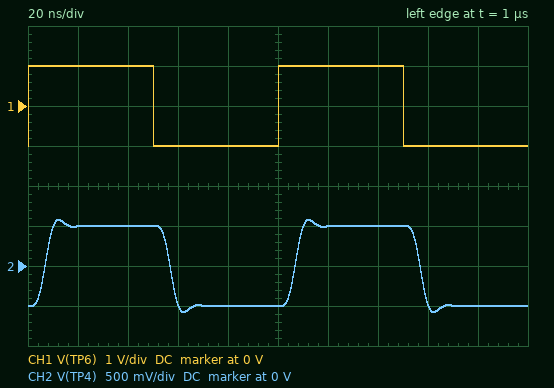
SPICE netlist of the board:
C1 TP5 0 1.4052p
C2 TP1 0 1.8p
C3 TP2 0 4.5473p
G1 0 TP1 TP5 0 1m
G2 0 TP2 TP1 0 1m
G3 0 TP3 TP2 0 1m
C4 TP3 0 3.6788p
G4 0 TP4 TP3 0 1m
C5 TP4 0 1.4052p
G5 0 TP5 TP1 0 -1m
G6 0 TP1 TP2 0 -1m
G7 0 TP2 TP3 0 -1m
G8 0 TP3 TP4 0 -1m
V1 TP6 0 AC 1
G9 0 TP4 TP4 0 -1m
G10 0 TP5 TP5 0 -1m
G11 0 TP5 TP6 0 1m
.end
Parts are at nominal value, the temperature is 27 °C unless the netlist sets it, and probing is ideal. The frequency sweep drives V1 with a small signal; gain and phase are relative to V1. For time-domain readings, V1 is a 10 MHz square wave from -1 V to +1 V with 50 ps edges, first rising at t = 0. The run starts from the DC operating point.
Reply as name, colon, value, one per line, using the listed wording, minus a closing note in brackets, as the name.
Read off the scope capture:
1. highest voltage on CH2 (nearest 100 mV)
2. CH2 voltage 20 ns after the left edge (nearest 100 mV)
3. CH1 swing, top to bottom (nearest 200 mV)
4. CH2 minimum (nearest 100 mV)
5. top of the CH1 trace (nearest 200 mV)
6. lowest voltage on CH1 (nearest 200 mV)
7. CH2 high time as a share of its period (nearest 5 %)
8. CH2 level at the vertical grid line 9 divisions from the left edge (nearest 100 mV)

highest voltage on CH2: 600 mV
CH2 voltage 20 ns after the left edge: 500 mV
CH1 swing, top to bottom: 2.0 V
CH2 minimum: -600 mV
top of the CH1 trace: 1.0 V
lowest voltage on CH1: -1.0 V
CH2 high time as a share of its period: 50 %
CH2 level at the vertical grid line 9 divisions from the left edge: -500 mV
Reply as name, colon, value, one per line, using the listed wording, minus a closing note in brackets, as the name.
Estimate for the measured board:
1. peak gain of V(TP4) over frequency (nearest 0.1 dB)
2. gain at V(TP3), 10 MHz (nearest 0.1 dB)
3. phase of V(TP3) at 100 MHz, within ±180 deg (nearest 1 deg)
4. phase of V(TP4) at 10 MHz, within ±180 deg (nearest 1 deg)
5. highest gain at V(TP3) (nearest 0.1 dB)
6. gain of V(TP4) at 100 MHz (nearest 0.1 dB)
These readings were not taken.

peak gain of V(TP4) over frequency: -6.0 dB
gain at V(TP3), 10 MHz: -6.0 dB
phase of V(TP3) at 100 MHz, within ±180 deg: 140 deg
phase of V(TP4) at 10 MHz, within ±180 deg: -23 deg
highest gain at V(TP3): -5.9 dB
gain of V(TP4) at 100 MHz: -14.0 dB
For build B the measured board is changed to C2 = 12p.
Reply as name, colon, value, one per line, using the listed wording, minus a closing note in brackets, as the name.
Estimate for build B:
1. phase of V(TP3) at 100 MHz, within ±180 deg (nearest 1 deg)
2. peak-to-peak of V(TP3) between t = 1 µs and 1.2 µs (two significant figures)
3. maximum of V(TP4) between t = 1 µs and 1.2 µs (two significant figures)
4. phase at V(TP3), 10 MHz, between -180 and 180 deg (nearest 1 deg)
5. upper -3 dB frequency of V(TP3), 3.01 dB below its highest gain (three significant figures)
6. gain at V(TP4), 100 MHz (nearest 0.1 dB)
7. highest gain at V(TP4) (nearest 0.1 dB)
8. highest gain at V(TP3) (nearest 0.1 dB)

phase of V(TP3) at 100 MHz, within ±180 deg: 75 deg
peak-to-peak of V(TP3) between t = 1 µs and 1.2 µs: 1.0 V
maximum of V(TP4) between t = 1 µs and 1.2 µs: 500 mV
phase at V(TP3), 10 MHz, between -180 and 180 deg: -36 deg
upper -3 dB frequency of V(TP3), 3.01 dB below its highest gain: 37.1 MHz
gain at V(TP4), 100 MHz: -34.5 dB
highest gain at V(TP4): -6.0 dB
highest gain at V(TP3): -6.0 dB
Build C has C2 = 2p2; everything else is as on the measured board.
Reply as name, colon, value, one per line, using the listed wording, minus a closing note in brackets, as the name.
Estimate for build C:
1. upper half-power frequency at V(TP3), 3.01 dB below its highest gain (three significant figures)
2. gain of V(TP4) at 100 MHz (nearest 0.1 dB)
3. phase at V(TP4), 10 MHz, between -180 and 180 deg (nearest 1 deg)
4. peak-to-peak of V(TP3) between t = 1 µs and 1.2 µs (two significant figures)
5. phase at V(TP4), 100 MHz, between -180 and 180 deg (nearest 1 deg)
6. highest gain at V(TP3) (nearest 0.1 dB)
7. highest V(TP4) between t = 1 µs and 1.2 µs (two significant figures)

upper half-power frequency at V(TP3), 3.01 dB below its highest gain: 84.7 MHz
gain of V(TP4) at 100 MHz: -15.5 dB
phase at V(TP4), 10 MHz, between -180 and 180 deg: -24 deg
peak-to-peak of V(TP3) between t = 1 µs and 1.2 µs: 1.3 V
phase at V(TP4), 100 MHz, between -180 and 180 deg: 80 deg
highest gain at V(TP3): -5.8 dB
highest V(TP4) between t = 1 µs and 1.2 µs: 600 mV
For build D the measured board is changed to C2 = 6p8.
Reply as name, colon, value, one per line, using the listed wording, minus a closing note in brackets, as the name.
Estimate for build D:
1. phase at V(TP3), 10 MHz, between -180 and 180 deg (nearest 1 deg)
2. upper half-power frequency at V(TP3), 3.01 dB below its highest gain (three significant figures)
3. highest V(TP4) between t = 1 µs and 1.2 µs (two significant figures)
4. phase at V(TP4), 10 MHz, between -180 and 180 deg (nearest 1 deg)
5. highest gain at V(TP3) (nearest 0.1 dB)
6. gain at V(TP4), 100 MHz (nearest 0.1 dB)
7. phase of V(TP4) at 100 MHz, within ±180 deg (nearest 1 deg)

phase at V(TP3), 10 MHz, between -180 and 180 deg: -27 deg
upper half-power frequency at V(TP3), 3.01 dB below its highest gain: 58.1 MHz
highest V(TP4) between t = 1 µs and 1.2 µs: 590 mV
phase at V(TP4), 10 MHz, between -180 and 180 deg: -32 deg
highest gain at V(TP3): -6.0 dB
gain at V(TP4), 100 MHz: -28.7 dB
phase of V(TP4) at 100 MHz, within ±180 deg: 38 deg
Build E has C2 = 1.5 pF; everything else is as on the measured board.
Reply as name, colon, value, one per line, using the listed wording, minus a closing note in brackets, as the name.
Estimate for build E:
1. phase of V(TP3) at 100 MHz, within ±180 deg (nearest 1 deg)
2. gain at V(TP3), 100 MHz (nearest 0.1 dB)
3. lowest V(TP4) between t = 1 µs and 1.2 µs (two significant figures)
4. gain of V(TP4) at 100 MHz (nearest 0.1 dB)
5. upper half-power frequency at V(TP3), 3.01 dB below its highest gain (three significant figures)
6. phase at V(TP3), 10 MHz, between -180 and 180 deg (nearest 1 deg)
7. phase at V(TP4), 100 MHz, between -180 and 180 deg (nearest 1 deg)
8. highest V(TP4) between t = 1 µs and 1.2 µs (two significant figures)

phase of V(TP3) at 100 MHz, within ±180 deg: 157 deg
gain at V(TP3), 100 MHz: -11.0 dB
lowest V(TP4) between t = 1 µs and 1.2 µs: -550 mV
gain of V(TP4) at 100 MHz: -13.5 dB
upper half-power frequency at V(TP3), 3.01 dB below its highest gain: 85.1 MHz
phase at V(TP3), 10 MHz, between -180 and 180 deg: -18 deg
phase at V(TP4), 100 MHz, between -180 and 180 deg: 116 deg
highest V(TP4) between t = 1 µs and 1.2 µs: 550 mV
